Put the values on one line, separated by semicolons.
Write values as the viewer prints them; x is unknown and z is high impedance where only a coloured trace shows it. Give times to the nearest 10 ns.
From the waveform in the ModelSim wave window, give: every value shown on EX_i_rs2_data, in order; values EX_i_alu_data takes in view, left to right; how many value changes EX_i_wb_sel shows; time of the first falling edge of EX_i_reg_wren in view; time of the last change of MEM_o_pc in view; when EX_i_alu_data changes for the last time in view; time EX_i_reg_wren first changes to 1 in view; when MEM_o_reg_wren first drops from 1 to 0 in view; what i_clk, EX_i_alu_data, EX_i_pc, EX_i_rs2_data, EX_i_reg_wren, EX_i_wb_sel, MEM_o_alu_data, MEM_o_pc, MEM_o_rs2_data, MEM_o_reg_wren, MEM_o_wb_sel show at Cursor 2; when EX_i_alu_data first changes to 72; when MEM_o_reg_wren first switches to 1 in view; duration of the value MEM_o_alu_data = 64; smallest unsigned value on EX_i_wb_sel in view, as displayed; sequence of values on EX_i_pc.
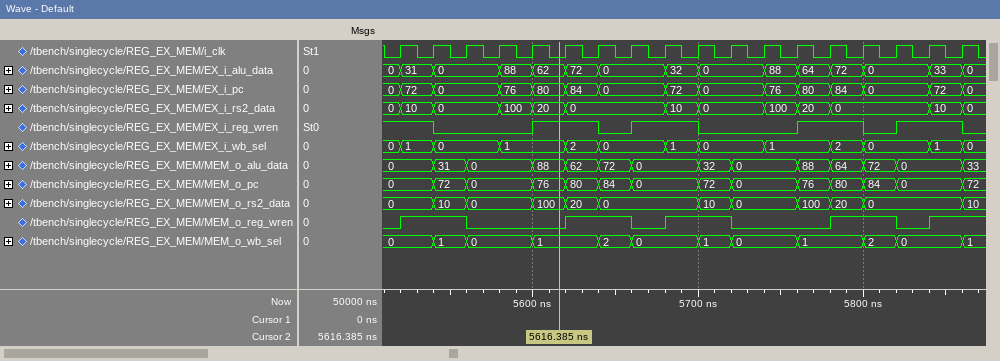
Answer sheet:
0, 10, 0, 100, 20, 0, 10, 0, 100, 20, 0, 10, 0; 0, 31, 0, 88, 62, 72, 0, 32, 0, 88, 64, 72, 0, 33, 0; 12; 5540 ns; 5860 ns; 5860 ns; 5600 ns; 5560 ns; i_clk=0, EX_i_alu_data=62, EX_i_pc=80, EX_i_rs2_data=20, EX_i_reg_wren=1, EX_i_wb_sel=1, MEM_o_alu_data=88, MEM_o_pc=76, MEM_o_rs2_data=100, MEM_o_reg_wren=0, MEM_o_wb_sel=1; 5620 ns; 5520 ns; 20 ns; 0; 0, 72, 0, 76, 80, 84, 0, 72, 0, 76, 80, 84, 0, 72, 0
